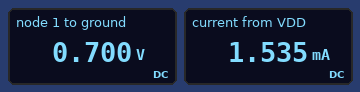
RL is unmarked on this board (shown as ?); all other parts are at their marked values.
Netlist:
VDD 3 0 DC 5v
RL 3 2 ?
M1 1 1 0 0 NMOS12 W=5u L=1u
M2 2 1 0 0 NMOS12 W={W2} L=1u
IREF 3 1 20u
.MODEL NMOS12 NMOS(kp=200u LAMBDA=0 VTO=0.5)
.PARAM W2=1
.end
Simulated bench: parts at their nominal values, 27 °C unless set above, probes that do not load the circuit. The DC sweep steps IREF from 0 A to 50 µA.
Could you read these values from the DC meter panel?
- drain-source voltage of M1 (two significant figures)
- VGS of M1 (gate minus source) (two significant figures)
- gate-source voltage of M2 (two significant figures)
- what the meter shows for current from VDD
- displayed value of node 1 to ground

700 mV
700 mV
700 mV
1.535 mA
0.700 V
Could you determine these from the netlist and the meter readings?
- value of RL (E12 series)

3.3 kΩ
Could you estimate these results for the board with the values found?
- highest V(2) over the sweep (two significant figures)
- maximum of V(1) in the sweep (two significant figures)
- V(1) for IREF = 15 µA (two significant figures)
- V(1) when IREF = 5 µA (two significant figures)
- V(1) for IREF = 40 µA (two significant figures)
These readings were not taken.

5.0 V
820 mV
670 mV
600 mV
780 mV
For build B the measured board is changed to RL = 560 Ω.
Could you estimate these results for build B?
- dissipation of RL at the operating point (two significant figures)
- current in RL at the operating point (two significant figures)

45 mW
8.9 mA
